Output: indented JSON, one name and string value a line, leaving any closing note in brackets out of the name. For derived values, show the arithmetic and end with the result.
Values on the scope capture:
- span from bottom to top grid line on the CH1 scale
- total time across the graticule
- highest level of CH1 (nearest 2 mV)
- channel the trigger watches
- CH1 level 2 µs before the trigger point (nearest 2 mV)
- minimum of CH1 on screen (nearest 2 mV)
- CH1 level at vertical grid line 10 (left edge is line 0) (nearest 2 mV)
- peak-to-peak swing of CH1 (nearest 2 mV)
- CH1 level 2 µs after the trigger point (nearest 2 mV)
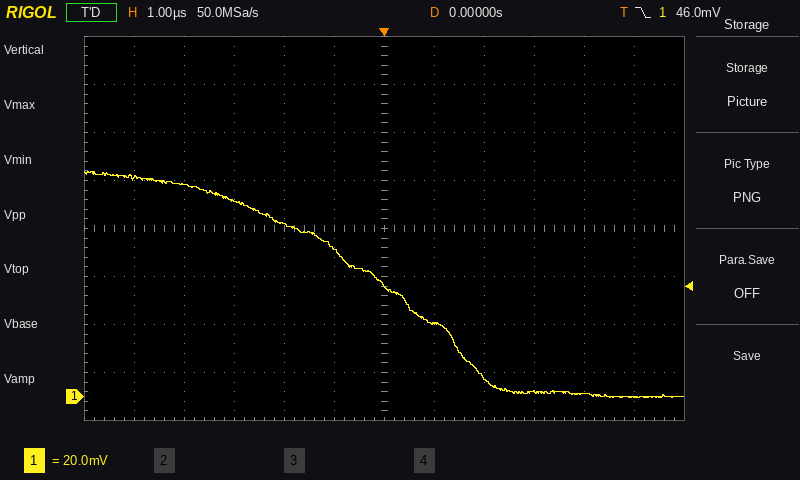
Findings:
{
  "span from bottom to top grid line on the CH1 scale": "160 mV",
  "total time across the graticule": "12 µs",
  "highest level of CH1": "94 mV",
  "channel the trigger watches": "CH1",
  "CH1 level 2 µs before the trigger point": "72 mV",
  "minimum of CH1 on screen": "0 mV",
  "CH1 level at vertical grid line 10 (left edge is line 0)": "2 mV",
  "peak-to-peak swing of CH1": "94 mV − (0 mV) = 94 mV",
  "CH1 level 2 µs after the trigger point": "8 mV"
}
